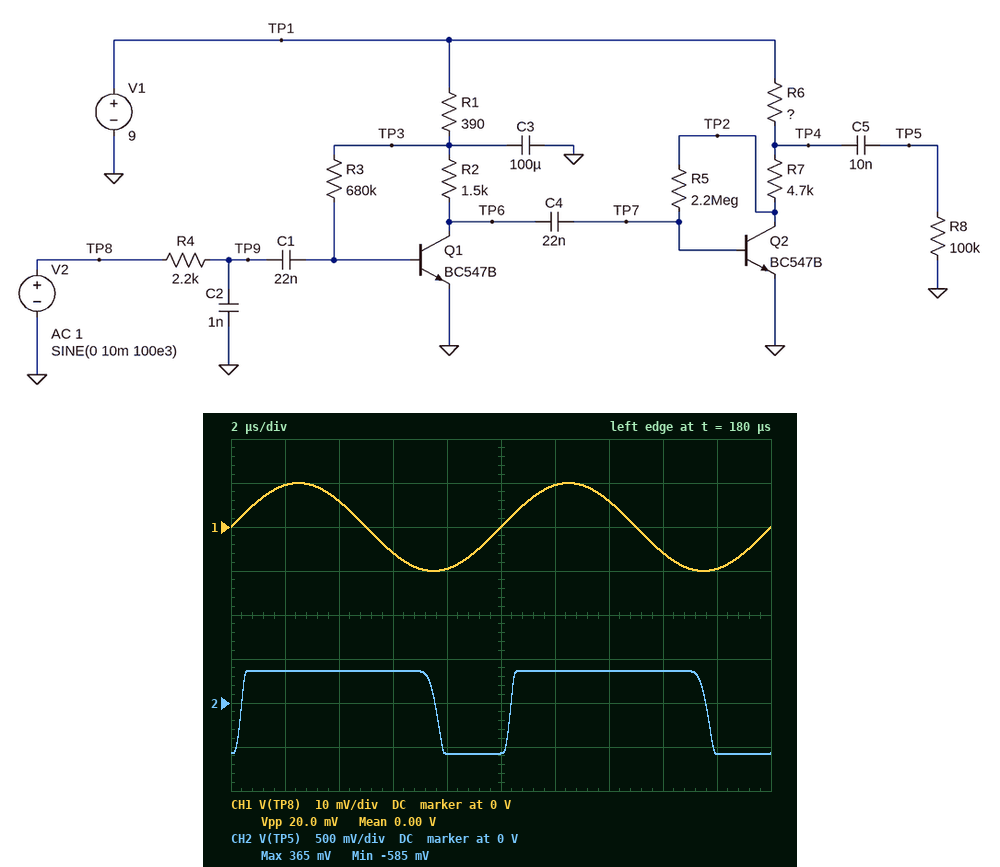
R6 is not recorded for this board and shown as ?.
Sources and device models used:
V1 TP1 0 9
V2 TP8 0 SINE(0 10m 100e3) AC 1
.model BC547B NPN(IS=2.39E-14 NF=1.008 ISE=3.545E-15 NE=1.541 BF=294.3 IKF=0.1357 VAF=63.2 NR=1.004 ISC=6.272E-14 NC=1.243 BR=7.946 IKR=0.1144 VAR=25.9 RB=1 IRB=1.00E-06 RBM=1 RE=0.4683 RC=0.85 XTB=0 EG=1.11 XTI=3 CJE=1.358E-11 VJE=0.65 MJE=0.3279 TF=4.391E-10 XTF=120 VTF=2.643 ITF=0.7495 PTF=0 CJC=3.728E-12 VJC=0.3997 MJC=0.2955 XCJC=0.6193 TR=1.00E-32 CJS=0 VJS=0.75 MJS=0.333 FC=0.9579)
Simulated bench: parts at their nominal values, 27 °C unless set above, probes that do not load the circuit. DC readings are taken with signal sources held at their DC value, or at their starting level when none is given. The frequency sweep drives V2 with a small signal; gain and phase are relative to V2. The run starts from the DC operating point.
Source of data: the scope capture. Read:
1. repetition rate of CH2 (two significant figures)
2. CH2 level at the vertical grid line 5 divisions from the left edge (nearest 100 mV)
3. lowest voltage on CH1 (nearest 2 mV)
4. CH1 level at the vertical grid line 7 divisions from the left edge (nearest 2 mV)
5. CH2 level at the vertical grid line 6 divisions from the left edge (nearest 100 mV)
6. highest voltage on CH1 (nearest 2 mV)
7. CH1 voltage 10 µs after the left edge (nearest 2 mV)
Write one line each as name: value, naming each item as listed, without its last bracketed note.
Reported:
repetition rate of CH2: 100 kHz
CH2 level at the vertical grid line 5 divisions from the left edge: -600 mV
lowest voltage on CH1: -10 mV
CH1 level at the vertical grid line 7 divisions from the left edge: 6 mV
CH2 level at the vertical grid line 6 divisions from the left edge: 400 mV
highest voltage on CH1: 10 mV
CH1 voltage 10 µs after the left edge: 0 V
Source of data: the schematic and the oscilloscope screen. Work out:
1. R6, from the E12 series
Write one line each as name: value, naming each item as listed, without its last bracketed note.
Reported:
R6, from the E12 series: 560 Ω
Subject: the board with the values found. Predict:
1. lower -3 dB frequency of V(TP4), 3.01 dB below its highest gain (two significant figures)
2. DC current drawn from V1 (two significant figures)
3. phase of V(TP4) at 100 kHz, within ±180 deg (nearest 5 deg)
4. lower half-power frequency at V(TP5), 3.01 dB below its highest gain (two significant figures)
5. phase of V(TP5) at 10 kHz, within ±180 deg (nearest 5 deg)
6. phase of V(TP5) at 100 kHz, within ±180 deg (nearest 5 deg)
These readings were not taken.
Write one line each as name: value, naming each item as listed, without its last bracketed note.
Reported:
lower -3 dB frequency of V(TP4), 3.01 dB below its highest gain: 1.8 kHz
DC current drawn from V1: 3.7 mA
phase of V(TP4) at 100 kHz, within ±180 deg: -55 deg
lower half-power frequency at V(TP5), 3.01 dB below its highest gain: 1.8 kHz
phase of V(TP5) at 10 kHz, within ±180 deg: 5 deg
phase of V(TP5) at 100 kHz, within ±180 deg: -55 deg
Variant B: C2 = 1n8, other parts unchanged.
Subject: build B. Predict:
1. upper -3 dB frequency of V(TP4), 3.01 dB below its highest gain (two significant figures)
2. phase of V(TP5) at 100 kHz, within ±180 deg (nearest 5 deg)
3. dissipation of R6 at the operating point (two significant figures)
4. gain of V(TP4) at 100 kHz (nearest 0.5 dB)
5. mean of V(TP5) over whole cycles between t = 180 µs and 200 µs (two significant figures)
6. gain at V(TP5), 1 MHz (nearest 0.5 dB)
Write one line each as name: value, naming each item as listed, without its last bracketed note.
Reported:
upper -3 dB frequency of V(TP4), 3.01 dB below its highest gain: 64 kHz
phase of V(TP5) at 100 kHz, within ±180 deg: -65 deg
dissipation of R6 at the operating point: 250 µW
gain of V(TP4) at 100 kHz: 53.0 dB
mean of V(TP5) over whole cycles between t = 180 µs and 200 µs: 97 mV
gain at V(TP5), 1 MHz: 28.5 dB
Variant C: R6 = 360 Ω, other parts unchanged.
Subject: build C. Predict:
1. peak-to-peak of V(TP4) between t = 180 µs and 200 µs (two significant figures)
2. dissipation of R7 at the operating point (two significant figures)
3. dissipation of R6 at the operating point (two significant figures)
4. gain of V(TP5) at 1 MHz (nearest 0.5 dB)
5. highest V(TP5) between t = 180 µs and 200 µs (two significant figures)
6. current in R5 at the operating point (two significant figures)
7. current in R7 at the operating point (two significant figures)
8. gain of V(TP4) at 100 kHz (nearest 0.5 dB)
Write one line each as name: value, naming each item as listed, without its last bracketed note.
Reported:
peak-to-peak of V(TP4) between t = 180 µs and 200 µs: 630 mV
dissipation of R7 at the operating point: 2.2 mW
dissipation of R6 at the operating point: 170 µW
gain of V(TP5) at 1 MHz: 29.5 dB
highest V(TP5) between t = 180 µs and 200 µs: 240 mV
current in R5 at the operating point: 2.2 µA
current in R7 at the operating point: 680 µA
gain of V(TP4) at 100 kHz: 52.0 dB
